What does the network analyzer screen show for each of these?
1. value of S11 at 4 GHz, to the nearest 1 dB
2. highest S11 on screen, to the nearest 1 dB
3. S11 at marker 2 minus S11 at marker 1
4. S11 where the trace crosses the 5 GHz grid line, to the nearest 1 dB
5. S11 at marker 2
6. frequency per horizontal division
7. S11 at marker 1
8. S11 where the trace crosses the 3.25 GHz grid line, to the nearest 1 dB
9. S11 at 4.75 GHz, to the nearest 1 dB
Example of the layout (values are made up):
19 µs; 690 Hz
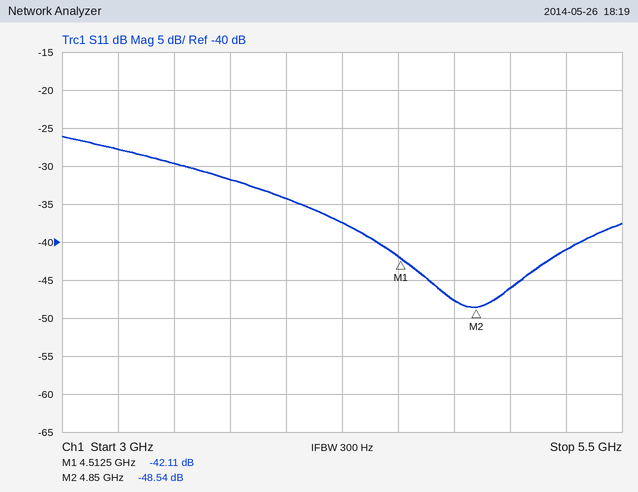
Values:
-34 dB; -26 dB; -6.43 dB; -46 dB; -48.54 dB; 250 MHz; -42.11 dB; -28 dB; -48 dB
